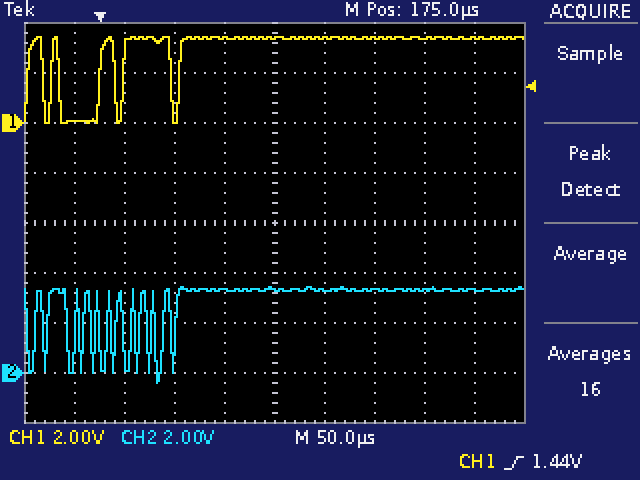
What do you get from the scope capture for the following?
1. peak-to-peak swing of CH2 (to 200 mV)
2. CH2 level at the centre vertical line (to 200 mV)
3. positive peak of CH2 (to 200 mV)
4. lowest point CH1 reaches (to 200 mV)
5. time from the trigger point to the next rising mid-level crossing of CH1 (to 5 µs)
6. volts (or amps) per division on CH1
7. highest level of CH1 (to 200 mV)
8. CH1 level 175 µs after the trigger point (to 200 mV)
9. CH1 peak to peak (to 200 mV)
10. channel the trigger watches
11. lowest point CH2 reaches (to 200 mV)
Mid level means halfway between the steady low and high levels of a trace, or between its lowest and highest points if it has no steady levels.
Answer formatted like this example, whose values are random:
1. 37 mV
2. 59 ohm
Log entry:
1. 3.8 V
2. 3.4 V
3. 3.4 V
4. 0.0 V
5. 25 µs
6. 2 V
7. 3.4 V
8. 3.4 V
9. 3.4 V
10. CH1
11. -400 mV
